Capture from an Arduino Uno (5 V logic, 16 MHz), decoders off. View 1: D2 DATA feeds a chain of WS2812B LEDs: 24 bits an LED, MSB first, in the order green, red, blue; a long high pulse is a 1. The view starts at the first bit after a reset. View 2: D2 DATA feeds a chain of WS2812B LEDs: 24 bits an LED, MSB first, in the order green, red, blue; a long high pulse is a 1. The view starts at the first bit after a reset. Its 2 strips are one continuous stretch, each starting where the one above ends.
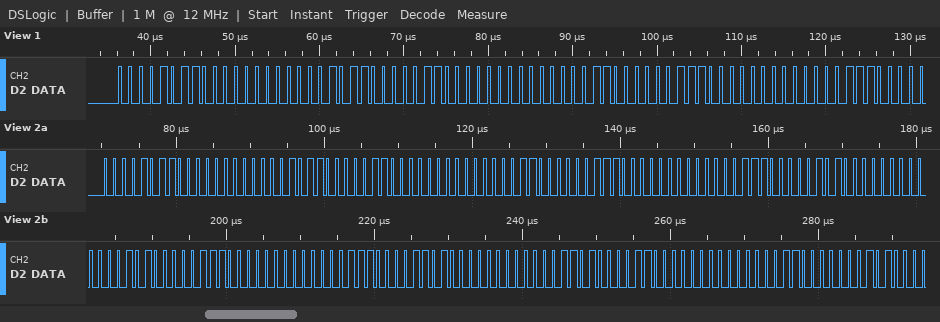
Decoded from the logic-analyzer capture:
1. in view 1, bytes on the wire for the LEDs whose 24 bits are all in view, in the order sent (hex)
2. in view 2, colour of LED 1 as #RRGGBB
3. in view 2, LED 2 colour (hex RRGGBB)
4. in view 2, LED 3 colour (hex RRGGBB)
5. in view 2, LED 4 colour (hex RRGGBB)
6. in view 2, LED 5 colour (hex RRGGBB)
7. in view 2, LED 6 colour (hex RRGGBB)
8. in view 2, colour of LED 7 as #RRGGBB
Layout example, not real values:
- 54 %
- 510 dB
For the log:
- 0B 00 0B 06 00 06 07 00 07
- #000B0B
- #000606
- #000707
- #000505
- #000707
- #000D0D
- #000C0C
